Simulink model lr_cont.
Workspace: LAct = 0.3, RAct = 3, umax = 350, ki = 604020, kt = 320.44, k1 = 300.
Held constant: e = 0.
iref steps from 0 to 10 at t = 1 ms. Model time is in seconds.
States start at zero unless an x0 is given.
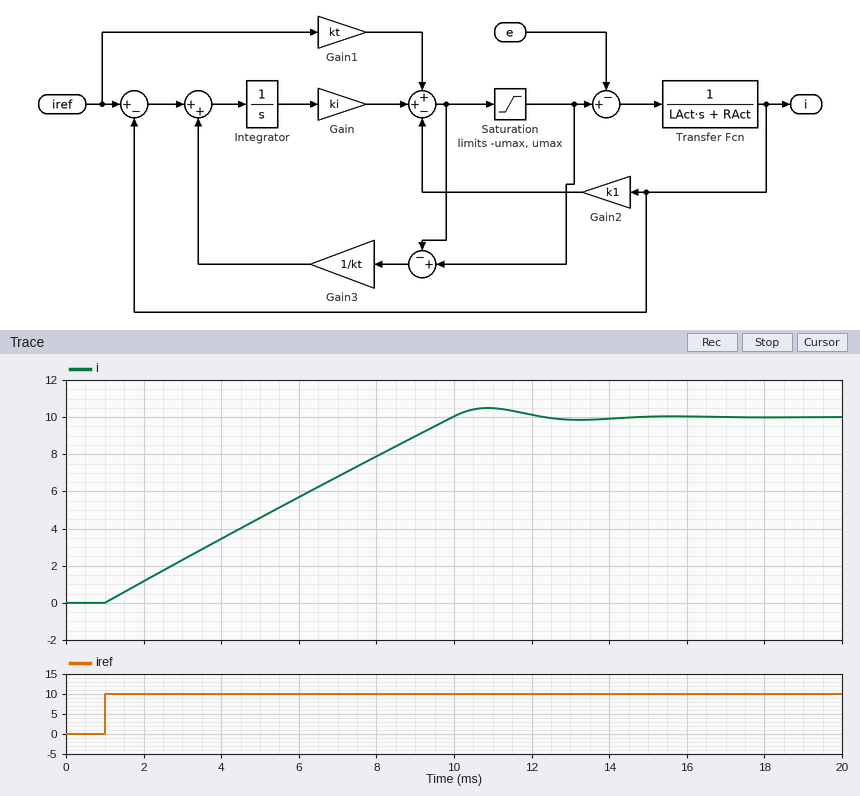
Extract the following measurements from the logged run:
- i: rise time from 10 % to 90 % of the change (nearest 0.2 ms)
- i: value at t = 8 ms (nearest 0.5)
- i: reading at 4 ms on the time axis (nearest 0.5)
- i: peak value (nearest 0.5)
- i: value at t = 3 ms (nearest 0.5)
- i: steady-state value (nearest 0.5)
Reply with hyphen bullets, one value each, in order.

- 7.2 ms
- 8.0
- 3.5
- 10.5
- 2.5
- 10.0
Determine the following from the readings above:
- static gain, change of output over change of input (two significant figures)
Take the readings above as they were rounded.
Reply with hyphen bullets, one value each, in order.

- 1.0
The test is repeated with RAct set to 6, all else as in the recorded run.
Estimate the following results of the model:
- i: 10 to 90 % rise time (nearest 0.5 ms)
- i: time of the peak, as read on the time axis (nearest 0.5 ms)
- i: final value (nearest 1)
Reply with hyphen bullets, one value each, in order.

- 7.5 ms
- 11.5 ms
- 10
